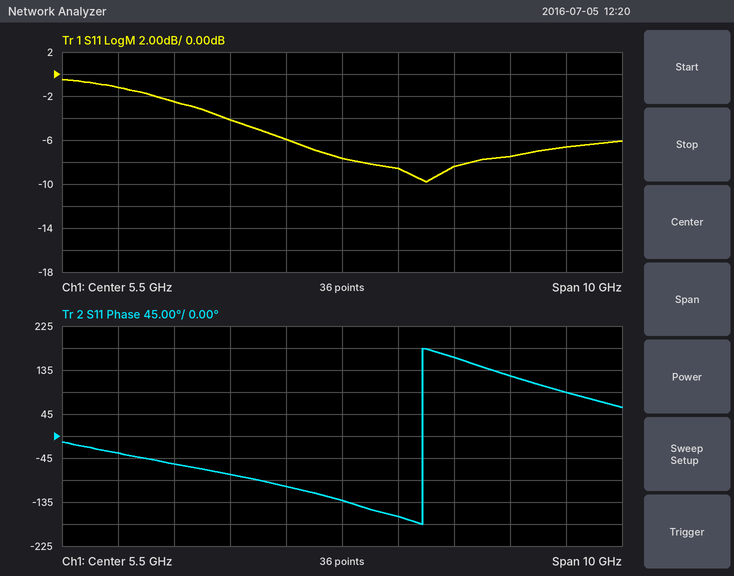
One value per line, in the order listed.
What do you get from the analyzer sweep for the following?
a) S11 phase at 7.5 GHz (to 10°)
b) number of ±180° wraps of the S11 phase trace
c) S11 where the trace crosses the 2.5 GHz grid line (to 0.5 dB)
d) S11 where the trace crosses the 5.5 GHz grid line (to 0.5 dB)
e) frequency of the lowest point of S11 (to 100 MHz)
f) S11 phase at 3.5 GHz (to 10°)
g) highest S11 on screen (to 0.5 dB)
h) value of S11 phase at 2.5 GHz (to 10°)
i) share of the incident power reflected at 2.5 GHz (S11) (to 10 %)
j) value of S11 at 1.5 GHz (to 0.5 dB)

160°
1
-2.5 dB
-7.5 dB
7.0 GHz
-80°
-0.5 dB
-60°
60 %
-1.0 dB
